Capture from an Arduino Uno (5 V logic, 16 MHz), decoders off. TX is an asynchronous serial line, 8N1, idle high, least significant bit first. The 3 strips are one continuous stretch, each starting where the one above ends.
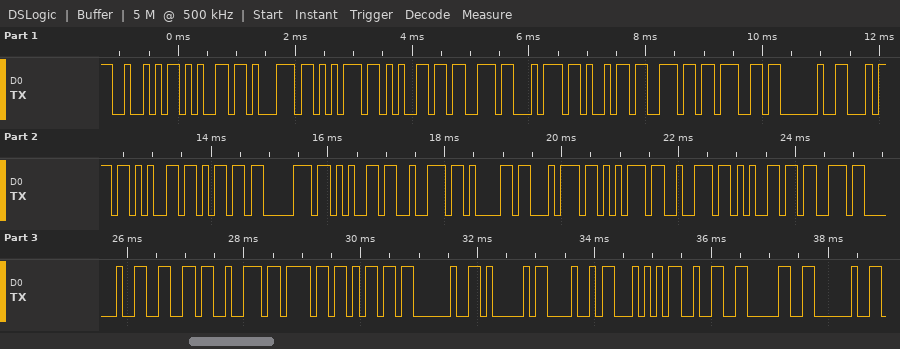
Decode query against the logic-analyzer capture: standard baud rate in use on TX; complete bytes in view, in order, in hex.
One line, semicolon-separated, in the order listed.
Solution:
9600 baud; 52 65 71 75 65 73 74 69 6E 67 20 74 65 6D 70 65 72 61 74 75 72 65 73 20 66 72 6F 6D 20 41 48 54 32 30 20
